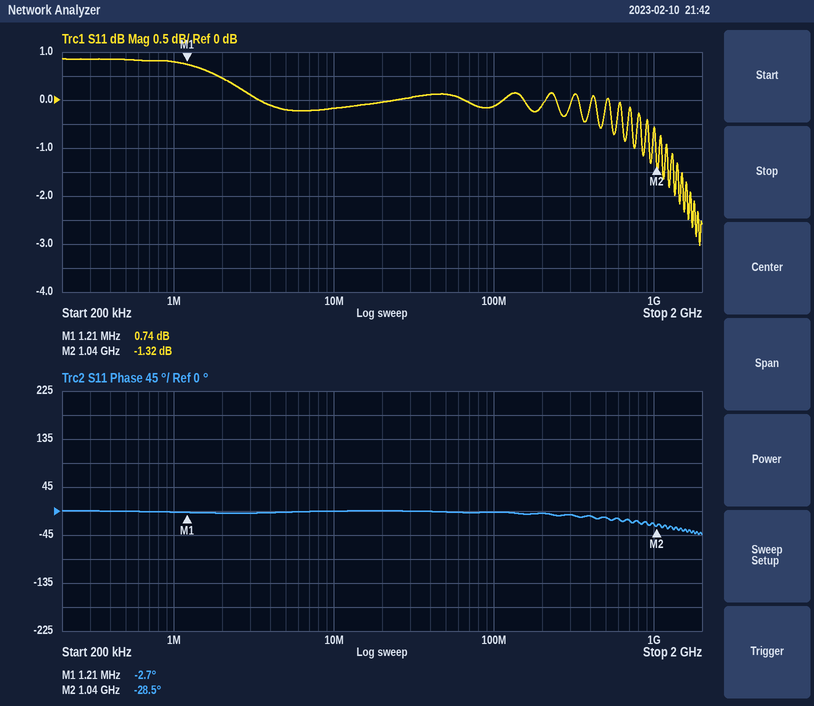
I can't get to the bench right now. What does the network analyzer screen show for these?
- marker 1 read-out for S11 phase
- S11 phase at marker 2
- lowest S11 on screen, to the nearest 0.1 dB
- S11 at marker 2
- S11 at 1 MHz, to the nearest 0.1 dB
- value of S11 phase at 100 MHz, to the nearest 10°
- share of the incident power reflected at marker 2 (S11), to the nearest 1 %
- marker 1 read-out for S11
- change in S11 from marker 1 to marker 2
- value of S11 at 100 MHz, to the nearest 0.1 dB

-2.7°
-28.5°
-3.0 dB
-1.32 dB
0.8 dB
0°
74 %
0.74 dB
-2.06 dB
-0.1 dB
